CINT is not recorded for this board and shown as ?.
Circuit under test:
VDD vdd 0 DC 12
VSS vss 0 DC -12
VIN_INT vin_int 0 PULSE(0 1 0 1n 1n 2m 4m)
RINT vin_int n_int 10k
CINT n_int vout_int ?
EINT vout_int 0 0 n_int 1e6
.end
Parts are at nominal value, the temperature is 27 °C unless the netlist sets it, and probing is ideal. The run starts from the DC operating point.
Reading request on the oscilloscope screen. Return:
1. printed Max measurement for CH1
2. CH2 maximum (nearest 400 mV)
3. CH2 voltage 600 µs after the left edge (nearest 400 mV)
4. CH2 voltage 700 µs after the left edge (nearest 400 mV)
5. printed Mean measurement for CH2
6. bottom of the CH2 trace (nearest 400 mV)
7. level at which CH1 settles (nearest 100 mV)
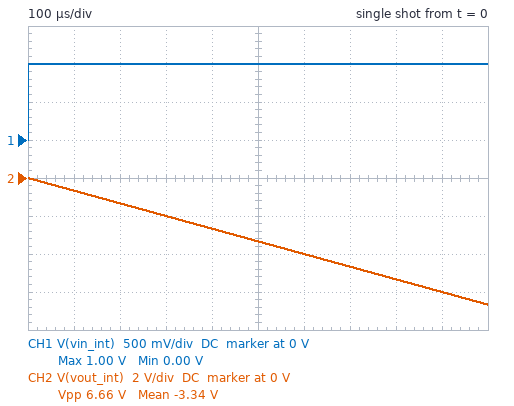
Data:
1.00 V
0 V
-4.0 V
-4.8 V
-3.34 V
-6.8 V
1.0 V
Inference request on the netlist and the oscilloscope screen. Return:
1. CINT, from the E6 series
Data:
15 nF
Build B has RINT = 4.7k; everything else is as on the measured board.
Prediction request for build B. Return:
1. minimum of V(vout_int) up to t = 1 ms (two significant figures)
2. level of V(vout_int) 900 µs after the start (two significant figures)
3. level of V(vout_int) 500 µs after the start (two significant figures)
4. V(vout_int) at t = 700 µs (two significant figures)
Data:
-14 V
-13 V
-7.1 V
-9.9 V
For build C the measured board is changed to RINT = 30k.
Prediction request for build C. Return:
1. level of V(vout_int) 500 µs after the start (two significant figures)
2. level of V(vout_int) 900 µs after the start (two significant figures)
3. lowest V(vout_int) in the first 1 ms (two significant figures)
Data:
-1.1 V
-2.0 V
-2.2 V
